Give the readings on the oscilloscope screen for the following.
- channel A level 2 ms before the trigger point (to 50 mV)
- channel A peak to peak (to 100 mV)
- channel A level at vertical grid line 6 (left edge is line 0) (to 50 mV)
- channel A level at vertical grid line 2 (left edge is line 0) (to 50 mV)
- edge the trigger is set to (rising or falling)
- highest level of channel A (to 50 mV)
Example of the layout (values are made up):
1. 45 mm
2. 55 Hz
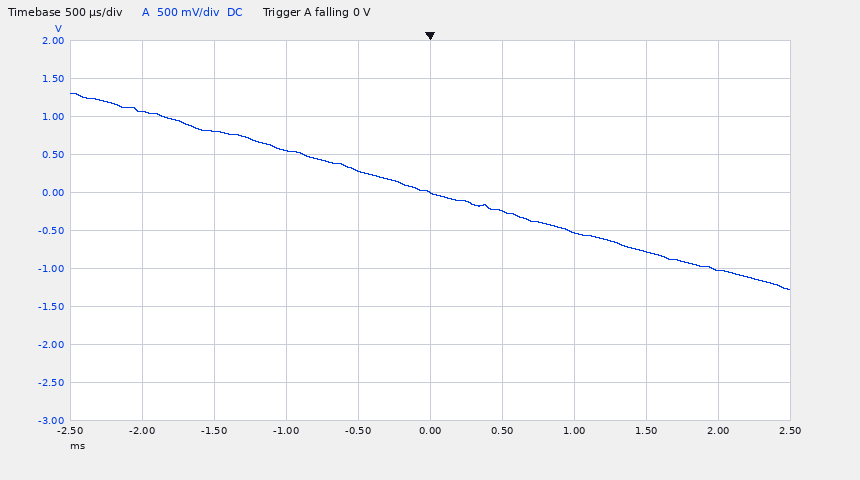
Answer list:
1. 1.05 V
2. 2.60 V
3. -250 mV
4. 800 mV
5. falling
6. 1.30 V
